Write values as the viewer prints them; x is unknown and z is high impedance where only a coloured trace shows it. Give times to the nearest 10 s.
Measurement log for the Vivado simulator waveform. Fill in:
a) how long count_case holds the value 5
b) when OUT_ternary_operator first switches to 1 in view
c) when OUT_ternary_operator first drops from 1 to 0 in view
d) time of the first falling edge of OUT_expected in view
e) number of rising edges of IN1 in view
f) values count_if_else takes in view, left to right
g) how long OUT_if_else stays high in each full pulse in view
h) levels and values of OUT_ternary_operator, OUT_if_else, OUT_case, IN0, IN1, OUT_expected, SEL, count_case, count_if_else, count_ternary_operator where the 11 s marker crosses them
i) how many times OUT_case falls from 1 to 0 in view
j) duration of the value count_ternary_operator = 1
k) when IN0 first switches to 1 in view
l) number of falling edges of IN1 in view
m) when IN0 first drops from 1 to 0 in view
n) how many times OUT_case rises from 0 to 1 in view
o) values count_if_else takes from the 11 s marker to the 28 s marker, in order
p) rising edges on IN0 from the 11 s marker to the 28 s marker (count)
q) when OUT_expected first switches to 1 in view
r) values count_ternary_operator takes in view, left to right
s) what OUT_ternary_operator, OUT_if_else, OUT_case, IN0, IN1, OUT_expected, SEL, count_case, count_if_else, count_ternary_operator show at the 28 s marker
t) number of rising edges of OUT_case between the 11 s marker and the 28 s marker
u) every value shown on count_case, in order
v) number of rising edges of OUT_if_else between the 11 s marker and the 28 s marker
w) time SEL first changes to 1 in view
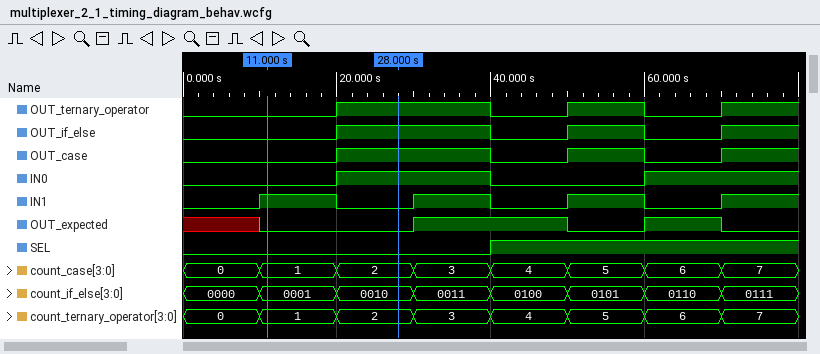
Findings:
10 s
20 s
40 s
50 s
4
0000, 0001, 0010, 0011, 0100, 0101, 0110, 0111
20 s, 10 s
OUT_ternary_operator=0, OUT_if_else=0, OUT_case=0, IN0=0, IN1=1, OUT_expected=0, SEL=0, count_case=1, count_if_else=0001, count_ternary_operator=1
2
10 s
20 s
3
40 s
3
0001, 0010
1
30 s
0, 1, 2, 3, 4, 5, 6, 7
OUT_ternary_operator=1, OUT_if_else=1, OUT_case=1, IN0=1, IN1=0, OUT_expected=0, SEL=0, count_case=2, count_if_else=0010, count_ternary_operator=2
1
0, 1, 2, 3, 4, 5, 6, 7
1
40 s
